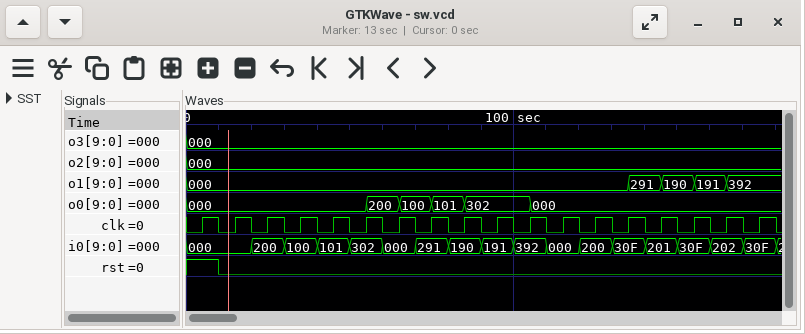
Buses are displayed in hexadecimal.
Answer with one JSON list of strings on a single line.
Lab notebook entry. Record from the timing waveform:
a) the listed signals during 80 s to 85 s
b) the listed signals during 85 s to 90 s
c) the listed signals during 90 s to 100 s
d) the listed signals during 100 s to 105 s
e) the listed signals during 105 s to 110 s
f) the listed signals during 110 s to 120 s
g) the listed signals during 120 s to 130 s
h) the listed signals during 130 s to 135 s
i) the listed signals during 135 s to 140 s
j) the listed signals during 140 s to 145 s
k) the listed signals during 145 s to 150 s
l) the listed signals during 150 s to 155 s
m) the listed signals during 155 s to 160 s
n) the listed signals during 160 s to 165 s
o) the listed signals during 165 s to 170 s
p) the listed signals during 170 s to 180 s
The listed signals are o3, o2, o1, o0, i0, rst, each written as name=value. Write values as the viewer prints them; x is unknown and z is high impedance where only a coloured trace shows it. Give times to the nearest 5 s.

["o3=000, o2=000, o1=000, o0=101, i0=190, rst=0", "o3=000, o2=000, o1=000, o0=302, i0=190, rst=0", "o3=000, o2=000, o1=000, o0=302, i0=191, rst=0", "o3=000, o2=000, o1=000, o0=302, i0=392, rst=0", "o3=000, o2=000, o1=000, o0=000, i0=392, rst=0", "o3=000, o2=000, o1=000, o0=000, i0=000, rst=0", "o3=000, o2=000, o1=000, o0=000, i0=200, rst=0", "o3=000, o2=000, o1=000, o0=000, i0=30F, rst=0", "o3=000, o2=000, o1=291, o0=000, i0=30F, rst=0", "o3=000, o2=000, o1=291, o0=000, i0=201, rst=0", "o3=000, o2=000, o1=190, o0=000, i0=201, rst=0", "o3=000, o2=000, o1=190, o0=000, i0=30F, rst=0", "o3=000, o2=000, o1=191, o0=000, i0=30F, rst=0", "o3=000, o2=000, o1=191, o0=000, i0=202, rst=0", "o3=000, o2=000, o1=392, o0=000, i0=202, rst=0", "o3=000, o2=000, o1=392, o0=000, i0=30F, rst=0"]
